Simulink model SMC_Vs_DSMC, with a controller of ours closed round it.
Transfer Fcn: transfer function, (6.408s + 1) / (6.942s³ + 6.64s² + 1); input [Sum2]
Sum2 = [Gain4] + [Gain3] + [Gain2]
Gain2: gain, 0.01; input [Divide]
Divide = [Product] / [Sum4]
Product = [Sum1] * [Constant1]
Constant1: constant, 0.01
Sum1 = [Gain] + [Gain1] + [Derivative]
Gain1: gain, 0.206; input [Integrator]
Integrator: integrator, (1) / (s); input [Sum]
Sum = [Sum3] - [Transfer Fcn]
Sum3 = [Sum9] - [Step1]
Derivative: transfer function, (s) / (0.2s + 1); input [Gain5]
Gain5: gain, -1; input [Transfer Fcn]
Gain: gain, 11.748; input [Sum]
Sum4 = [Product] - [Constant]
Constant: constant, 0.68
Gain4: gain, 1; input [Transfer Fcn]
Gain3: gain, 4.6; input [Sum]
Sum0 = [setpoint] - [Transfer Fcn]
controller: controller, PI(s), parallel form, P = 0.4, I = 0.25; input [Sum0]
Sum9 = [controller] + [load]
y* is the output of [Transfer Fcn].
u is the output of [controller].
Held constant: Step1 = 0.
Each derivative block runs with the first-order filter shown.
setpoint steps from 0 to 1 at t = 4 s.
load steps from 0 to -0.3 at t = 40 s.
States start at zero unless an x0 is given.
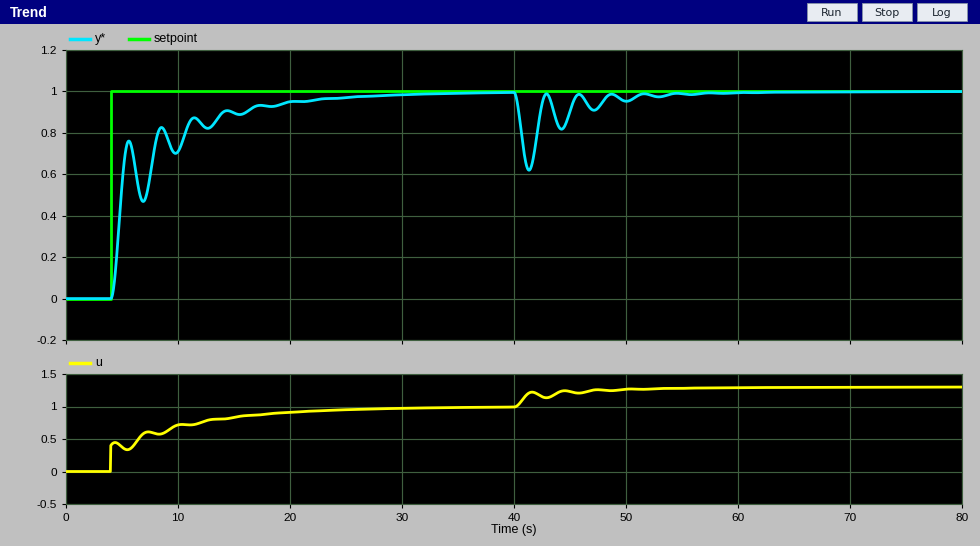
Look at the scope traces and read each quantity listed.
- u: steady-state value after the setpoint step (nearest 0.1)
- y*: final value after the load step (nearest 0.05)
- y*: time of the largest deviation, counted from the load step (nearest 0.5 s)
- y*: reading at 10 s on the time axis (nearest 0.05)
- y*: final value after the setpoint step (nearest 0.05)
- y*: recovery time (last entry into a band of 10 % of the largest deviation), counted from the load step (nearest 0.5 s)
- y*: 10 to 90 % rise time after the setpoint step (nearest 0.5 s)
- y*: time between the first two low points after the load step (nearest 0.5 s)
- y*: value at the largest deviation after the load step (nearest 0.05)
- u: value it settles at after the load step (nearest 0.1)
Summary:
1.0
1.00
1.5 s
0.70
1.00
10.5 s
9.5 s
3.0 s
0.60
1.3
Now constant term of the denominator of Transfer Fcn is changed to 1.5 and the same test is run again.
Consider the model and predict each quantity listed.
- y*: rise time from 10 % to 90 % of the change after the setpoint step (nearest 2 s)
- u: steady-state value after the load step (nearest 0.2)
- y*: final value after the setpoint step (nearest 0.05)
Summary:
12 s
1.4
1.00
